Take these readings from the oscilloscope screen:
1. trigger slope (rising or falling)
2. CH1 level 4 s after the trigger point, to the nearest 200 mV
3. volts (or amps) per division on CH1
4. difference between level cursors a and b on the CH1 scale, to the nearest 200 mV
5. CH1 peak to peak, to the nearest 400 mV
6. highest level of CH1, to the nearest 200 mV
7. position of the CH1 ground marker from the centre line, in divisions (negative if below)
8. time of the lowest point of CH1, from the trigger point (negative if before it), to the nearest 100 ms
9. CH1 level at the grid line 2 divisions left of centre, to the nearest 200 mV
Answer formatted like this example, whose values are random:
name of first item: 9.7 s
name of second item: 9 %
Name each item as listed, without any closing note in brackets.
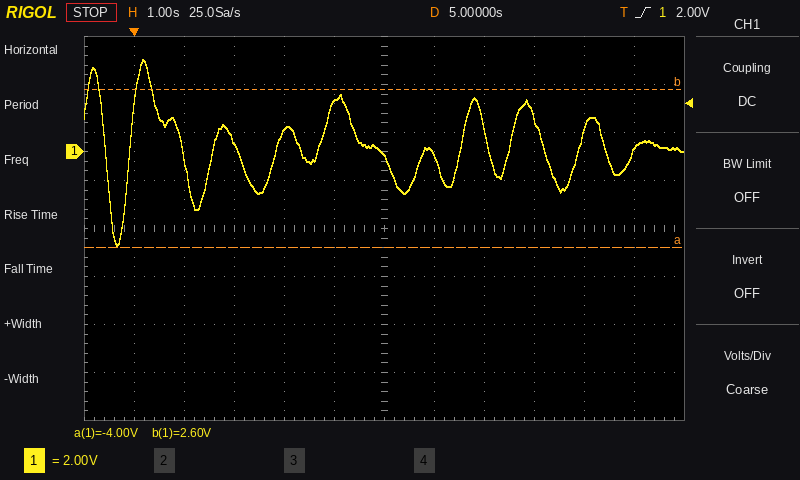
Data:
trigger slope: rising
CH1 level 4 s after the trigger point, to the nearest 200 mV: 2.0 V
volts (or amps) per division on CH1: 2 V
difference between level cursors a and b on the CH1 scale, to the nearest 200 mV: 6.6 V
CH1 peak to peak, to the nearest 400 mV: 7.6 V
highest level of CH1, to the nearest 200 mV: 3.8 V
position of the CH1 ground marker from the centre line, in divisions: +1.6 div
time of the lowest point of CH1, from the trigger point (negative if before it), to the nearest 100 ms: -300 ms
CH1 level at the grid line 2 divisions left of centre, to the nearest 200 mV: 800 mV
